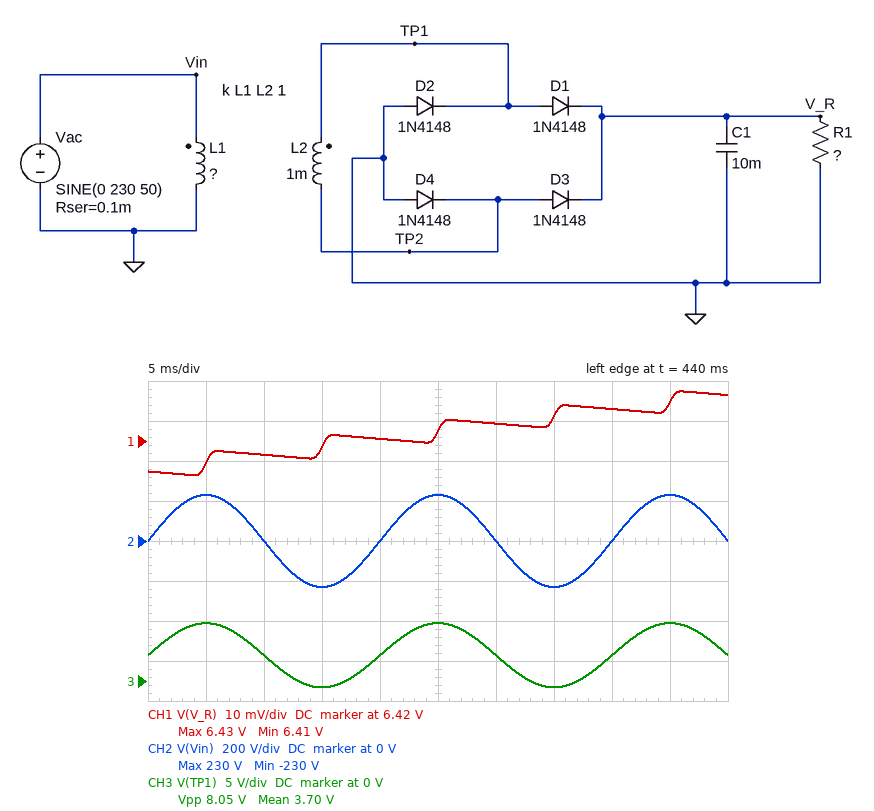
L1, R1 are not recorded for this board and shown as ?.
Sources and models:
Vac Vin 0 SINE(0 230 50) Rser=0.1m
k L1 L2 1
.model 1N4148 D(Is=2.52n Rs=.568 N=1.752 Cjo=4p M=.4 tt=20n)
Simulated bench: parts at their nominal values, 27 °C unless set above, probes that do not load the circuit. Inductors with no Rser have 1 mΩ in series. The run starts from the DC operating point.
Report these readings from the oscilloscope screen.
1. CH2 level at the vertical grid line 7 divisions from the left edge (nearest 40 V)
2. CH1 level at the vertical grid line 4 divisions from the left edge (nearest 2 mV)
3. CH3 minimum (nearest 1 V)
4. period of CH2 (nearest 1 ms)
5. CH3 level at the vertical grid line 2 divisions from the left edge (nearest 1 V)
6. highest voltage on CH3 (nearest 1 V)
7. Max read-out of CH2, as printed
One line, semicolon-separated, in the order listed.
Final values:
-240 V; 6.420 V; -1 V; 20 ms; 3 V; 7 V; 230 V
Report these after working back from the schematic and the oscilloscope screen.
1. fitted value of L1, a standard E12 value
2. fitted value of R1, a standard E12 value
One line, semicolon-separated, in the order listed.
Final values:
820 mH; 2.7 kΩ
